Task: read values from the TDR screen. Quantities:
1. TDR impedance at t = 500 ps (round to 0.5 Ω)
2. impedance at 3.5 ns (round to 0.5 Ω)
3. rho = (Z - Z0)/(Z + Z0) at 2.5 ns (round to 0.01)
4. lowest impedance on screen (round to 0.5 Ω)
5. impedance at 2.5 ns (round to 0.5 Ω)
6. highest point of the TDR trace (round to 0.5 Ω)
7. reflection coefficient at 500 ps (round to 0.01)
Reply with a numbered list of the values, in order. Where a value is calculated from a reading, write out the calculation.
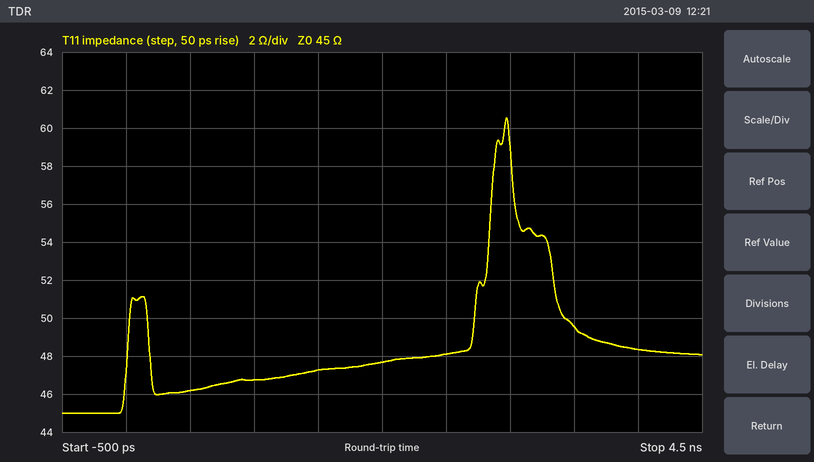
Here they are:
1. 46.0 Ω
2. 49.5 Ω
3. (48 − 45)/(48 + 45) ≈ +0.03
4. 45.0 Ω
5. 48.0 Ω
6. 60.5 Ω
7. (46 − 45)/(46 + 45) ≈ +0.01
